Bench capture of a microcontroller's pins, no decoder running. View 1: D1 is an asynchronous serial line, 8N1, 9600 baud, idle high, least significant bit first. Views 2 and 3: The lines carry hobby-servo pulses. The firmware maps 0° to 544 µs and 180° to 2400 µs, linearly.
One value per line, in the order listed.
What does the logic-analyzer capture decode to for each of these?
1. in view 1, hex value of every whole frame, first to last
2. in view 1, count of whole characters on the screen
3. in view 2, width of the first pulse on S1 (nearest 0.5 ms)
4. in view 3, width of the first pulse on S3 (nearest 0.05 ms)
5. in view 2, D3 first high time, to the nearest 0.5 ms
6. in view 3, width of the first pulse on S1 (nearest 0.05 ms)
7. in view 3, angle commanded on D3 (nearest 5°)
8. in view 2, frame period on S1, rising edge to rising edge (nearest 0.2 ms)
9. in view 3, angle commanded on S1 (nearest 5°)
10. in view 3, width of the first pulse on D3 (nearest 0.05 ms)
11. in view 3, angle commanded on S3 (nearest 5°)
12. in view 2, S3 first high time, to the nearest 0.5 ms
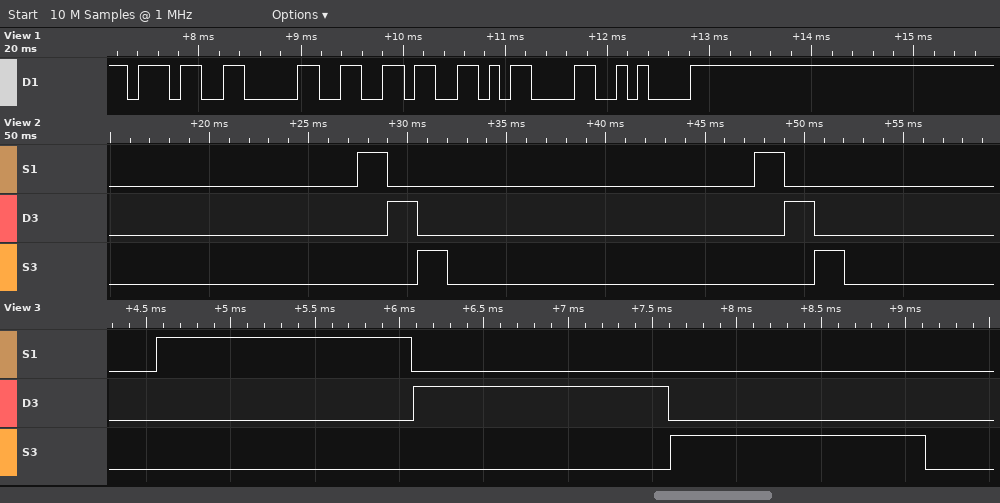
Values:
0x37 0x30 0x36 0x0D 0x0A
5
1.5 ms
1.50 ms
1.5 ms
1.50 ms
95°
20.0 ms
95°
1.50 ms
95°
1.5 ms
